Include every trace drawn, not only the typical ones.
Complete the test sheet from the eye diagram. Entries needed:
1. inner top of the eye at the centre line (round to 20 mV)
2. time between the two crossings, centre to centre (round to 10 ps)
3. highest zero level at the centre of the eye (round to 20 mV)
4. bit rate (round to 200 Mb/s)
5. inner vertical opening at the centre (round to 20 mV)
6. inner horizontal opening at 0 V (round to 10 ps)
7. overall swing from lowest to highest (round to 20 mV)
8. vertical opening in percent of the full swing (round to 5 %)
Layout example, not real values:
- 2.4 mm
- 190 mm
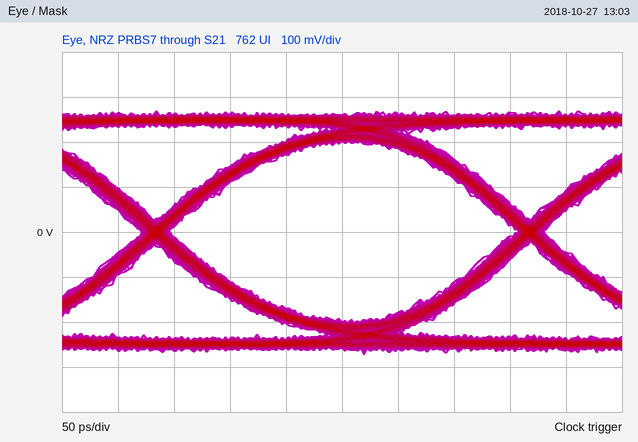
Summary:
- 200 mV
- 330 ps
- -200 mV
- 3.0 Gb/s
- 400 mV
- 310 ps
- 540 mV
- 75 %
